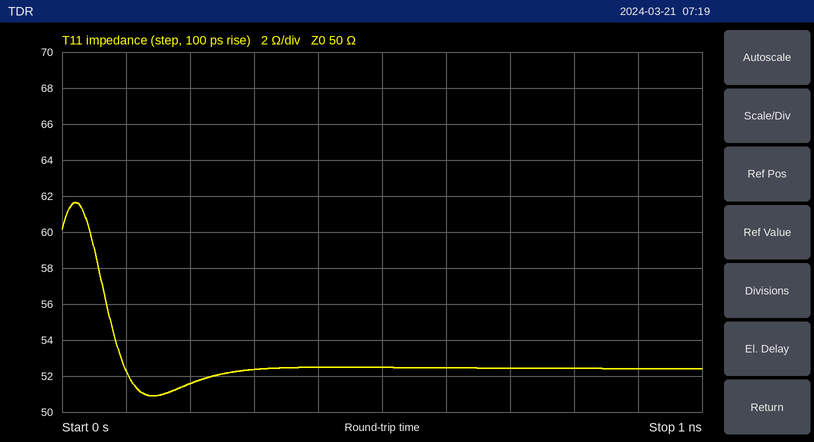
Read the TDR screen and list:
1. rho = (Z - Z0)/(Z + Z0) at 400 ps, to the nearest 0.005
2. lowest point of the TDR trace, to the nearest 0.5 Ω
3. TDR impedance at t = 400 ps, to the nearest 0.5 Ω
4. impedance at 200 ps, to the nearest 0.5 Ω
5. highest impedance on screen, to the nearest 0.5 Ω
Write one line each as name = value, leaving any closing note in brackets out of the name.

rho = (Z - Z0)/(Z + Z0) at 400 ps, to the nearest 0.005 = +0.025
lowest point of the TDR trace, to the nearest 0.5 Ω = 51.0 Ω
TDR impedance at t = 400 ps, to the nearest 0.5 Ω = 52.5 Ω
impedance at 200 ps, to the nearest 0.5 Ω = 51.5 Ω
highest impedance on screen, to the nearest 0.5 Ω = 61.5 Ω
